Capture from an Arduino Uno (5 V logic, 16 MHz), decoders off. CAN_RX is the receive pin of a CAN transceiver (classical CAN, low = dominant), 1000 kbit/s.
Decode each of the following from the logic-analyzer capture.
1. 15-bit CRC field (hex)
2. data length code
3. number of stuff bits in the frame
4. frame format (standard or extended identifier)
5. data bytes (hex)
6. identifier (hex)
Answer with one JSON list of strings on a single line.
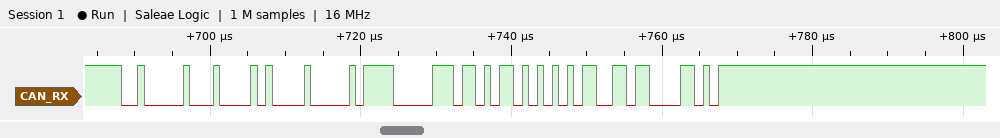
["0x4D86", "5", "3", "standard", "08 1E 0D AD 55", "0x201"]
